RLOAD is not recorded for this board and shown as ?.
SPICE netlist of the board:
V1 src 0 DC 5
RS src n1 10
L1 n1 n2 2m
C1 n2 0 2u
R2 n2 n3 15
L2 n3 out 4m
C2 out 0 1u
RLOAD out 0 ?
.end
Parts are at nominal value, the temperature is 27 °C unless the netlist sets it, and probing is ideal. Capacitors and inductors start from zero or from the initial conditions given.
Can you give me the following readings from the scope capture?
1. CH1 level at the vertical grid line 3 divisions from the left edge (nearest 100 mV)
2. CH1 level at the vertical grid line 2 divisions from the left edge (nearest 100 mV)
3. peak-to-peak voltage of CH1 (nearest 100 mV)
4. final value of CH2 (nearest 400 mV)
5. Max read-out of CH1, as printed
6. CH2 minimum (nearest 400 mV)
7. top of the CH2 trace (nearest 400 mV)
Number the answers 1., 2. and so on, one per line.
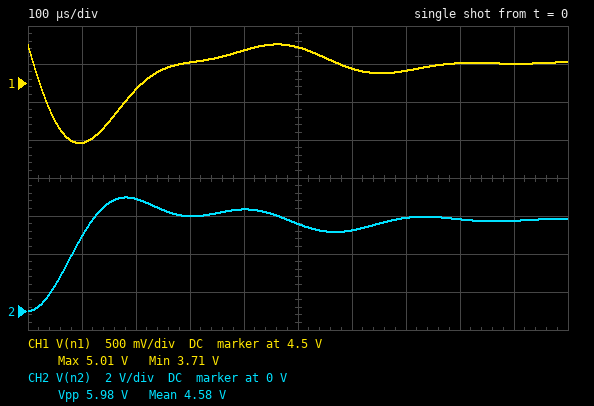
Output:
1. 4.8 V
2. 4.4 V
3. 1.3 V
4. 4.8 V
5. 5.01 V
6. 0 V
7. 6.0 V
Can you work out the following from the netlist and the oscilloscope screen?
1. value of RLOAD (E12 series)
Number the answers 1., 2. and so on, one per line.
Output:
1. 180 Ω
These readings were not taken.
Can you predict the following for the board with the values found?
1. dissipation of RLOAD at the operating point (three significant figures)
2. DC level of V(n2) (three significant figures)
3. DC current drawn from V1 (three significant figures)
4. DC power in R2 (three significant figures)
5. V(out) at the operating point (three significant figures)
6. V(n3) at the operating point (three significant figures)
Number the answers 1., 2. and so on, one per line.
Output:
1. 107 mW
2. 4.76 V
3. 24.4 mA
4. 8.92 mW
5. 4.39 V
6. 4.39 V
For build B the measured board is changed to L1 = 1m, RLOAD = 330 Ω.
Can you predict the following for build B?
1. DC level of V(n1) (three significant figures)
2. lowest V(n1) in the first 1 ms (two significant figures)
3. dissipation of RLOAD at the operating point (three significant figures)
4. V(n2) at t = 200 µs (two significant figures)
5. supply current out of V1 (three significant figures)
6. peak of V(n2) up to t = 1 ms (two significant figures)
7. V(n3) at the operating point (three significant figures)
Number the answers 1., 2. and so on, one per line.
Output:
1. 4.86 V
2. 3.3 V
3. 65.5 mW
4. 4.6 V
5. 14.1 mA
6. 6.1 V
7. 4.65 V
